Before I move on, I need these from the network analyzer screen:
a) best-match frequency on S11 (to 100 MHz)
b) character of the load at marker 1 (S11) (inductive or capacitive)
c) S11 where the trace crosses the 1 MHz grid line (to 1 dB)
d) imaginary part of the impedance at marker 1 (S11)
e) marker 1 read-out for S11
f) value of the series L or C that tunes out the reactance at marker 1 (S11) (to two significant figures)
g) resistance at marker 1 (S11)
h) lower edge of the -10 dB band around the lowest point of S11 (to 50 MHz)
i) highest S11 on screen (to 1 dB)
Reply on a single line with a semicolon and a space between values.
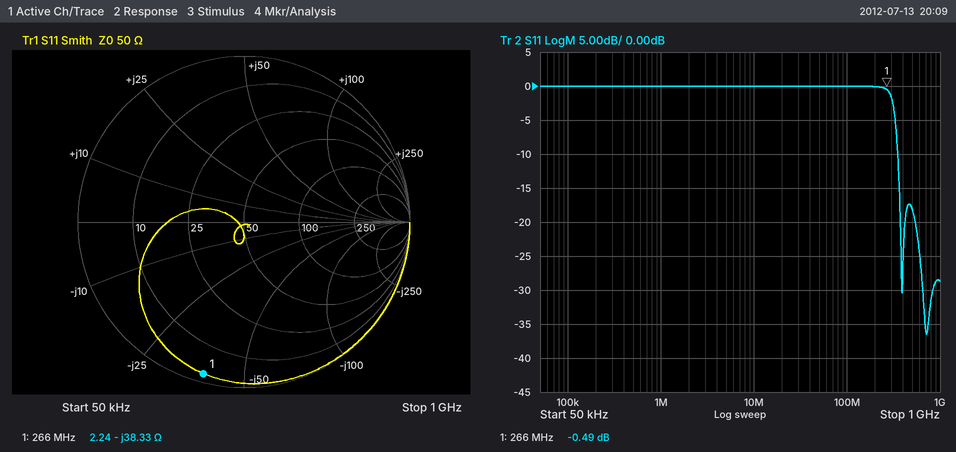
700 MHz; capacitive; 0 dB; -38.33 Ω; -0.49 dB; 23 nH; 2.24 Ω; 350 MHz; 0 dB
